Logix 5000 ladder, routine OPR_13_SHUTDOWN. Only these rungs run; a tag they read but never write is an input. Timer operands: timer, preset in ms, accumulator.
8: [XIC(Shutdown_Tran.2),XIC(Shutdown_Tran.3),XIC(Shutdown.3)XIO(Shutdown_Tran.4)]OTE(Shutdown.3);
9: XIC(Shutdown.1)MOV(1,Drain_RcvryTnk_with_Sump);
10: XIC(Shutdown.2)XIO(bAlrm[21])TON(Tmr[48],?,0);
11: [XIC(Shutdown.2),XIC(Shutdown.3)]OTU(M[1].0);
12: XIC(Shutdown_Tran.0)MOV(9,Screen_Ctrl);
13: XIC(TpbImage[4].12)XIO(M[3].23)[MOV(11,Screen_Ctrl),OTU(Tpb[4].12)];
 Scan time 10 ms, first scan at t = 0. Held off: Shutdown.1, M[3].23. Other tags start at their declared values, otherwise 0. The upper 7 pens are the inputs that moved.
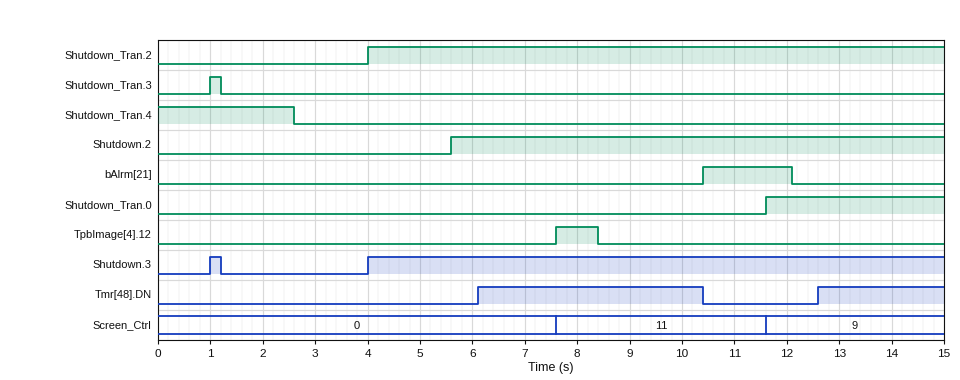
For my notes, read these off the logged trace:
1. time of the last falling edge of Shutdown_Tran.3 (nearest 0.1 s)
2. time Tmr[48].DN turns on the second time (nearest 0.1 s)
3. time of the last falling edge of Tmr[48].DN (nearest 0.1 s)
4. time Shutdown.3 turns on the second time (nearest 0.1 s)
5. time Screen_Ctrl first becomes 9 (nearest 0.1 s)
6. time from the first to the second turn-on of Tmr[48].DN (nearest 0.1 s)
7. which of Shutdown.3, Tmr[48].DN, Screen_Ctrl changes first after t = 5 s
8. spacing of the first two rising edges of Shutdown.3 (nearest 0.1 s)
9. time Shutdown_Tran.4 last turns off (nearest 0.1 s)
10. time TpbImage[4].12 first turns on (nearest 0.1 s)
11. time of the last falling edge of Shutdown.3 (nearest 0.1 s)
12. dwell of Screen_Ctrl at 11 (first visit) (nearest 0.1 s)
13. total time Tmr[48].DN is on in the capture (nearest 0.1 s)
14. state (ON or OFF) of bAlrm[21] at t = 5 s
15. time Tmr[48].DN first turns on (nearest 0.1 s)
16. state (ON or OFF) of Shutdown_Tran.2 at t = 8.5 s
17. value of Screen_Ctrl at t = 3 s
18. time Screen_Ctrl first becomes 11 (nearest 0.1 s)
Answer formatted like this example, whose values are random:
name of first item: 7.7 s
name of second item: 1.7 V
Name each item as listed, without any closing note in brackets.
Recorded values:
time of the last falling edge of Shutdown_Tran.3: 1.2 s
time Tmr[48].DN turns on the second time: 12.6 s
time of the last falling edge of Tmr[48].DN: 10.4 s
time Shutdown.3 turns on the second time: 4.0 s
time Screen_Ctrl first becomes 9: 11.6 s
time from the first to the second turn-on of Tmr[48].DN: 6.5 s
which of Shutdown.3, Tmr[48].DN, Screen_Ctrl changes first after t = 5 s: Tmr[48].DN
spacing of the first two rising edges of Shutdown.3: 3.0 s
time Shutdown_Tran.4 last turns off: 2.6 s
time TpbImage[4].12 first turns on: 7.6 s
time of the last falling edge of Shutdown.3: 1.2 s
dwell of Screen_Ctrl at 11 (first visit): 4.0 s
total time Tmr[48].DN is on in the capture: 6.7 s
state (ON or OFF) of bAlrm[21] at t = 5 s: OFF
time Tmr[48].DN first turns on: 6.1 s
state (ON or OFF) of Shutdown_Tran.2 at t = 8.5 s: ON
value of Screen_Ctrl at t = 3 s: 0
time Screen_Ctrl first becomes 11: 7.6 s
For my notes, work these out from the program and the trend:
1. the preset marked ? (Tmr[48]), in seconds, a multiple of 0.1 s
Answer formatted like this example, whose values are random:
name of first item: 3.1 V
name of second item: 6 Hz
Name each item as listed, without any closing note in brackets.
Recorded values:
the preset marked ? (Tmr[48]), in seconds, a multiple of 0.1 s: 0.5 s
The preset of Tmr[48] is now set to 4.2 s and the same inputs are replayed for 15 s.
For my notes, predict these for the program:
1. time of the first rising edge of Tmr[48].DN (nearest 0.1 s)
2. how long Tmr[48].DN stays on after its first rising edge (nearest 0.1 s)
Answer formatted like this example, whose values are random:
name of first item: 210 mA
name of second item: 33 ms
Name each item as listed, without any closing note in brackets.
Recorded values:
time of the first rising edge of Tmr[48].DN: 9.8 s
how long Tmr[48].DN stays on after its first rising edge: 0.6 s
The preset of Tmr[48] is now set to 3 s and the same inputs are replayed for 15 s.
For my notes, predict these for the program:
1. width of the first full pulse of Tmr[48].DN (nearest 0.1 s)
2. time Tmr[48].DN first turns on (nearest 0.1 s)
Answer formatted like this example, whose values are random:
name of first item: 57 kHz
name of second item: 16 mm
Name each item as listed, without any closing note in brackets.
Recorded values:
width of the first full pulse of Tmr[48].DN: 1.8 s
time Tmr[48].DN first turns on: 8.6 s
